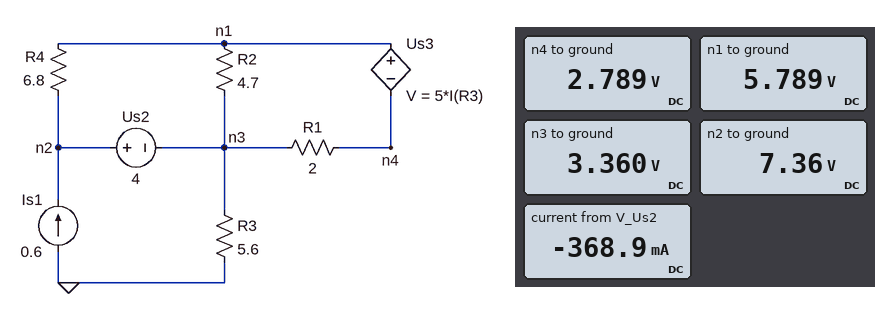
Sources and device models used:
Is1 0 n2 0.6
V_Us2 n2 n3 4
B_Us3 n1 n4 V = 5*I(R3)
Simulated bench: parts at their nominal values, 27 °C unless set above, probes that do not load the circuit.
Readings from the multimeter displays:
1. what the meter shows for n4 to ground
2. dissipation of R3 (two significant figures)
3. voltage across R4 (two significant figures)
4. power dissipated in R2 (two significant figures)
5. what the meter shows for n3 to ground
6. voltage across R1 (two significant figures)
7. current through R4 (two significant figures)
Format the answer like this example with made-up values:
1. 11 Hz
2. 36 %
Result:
1. 2.789 V
2. 2.0 W
3. 1.6 V
4. 1.3 W
5. 3.360 V
6. 570 mV
7. 230 mA
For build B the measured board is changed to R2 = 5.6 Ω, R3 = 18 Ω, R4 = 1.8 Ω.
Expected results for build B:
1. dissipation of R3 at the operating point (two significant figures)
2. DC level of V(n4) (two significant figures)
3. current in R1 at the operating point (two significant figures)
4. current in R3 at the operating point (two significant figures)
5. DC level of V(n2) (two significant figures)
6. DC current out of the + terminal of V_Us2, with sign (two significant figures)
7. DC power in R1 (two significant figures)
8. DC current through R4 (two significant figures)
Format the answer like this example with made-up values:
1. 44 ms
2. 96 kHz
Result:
1. 6.5 W
2. 11 V
3. 8.0 mA
4. 600 mA
5. 15 V
6. -53 mA
7. 130 µW
8. 550 mA
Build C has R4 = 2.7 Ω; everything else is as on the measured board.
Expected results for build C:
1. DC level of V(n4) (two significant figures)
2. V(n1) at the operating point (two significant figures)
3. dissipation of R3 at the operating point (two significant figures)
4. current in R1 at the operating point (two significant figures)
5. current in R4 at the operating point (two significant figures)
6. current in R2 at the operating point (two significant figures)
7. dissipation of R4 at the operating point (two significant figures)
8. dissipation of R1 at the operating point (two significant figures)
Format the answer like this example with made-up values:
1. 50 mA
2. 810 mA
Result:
1. 3.1 V
2. 6.1 V
3. 2.0 W
4. 120 mA
5. 460 mA
6. 590 mA
7. 580 mW
8. 31 mW
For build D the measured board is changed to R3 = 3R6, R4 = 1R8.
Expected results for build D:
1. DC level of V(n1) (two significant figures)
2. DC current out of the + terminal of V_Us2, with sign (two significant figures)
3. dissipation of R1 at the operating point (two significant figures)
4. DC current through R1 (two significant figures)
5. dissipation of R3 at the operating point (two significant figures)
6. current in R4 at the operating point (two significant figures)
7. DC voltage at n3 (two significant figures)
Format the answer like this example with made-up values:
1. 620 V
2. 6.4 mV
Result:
1. 5.1 V
2. -8.2 mA
3. 2.1 mW
4. 33 mA
5. 1.3 W
6. 590 mA
7. 2.2 V
